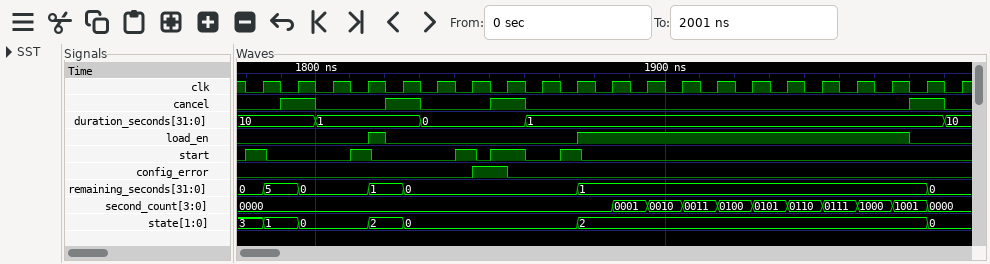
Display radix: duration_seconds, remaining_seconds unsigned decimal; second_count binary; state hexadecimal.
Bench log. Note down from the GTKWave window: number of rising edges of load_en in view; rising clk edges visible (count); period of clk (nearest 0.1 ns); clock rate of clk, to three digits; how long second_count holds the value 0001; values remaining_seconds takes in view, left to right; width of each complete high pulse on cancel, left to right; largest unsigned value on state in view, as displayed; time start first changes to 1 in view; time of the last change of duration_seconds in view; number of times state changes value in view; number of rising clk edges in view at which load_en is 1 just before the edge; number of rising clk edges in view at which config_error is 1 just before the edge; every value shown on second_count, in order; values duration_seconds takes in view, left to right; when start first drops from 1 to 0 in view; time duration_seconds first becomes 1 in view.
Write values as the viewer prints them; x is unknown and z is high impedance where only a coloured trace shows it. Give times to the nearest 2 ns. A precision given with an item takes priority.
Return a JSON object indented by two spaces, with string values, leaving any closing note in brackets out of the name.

{
  "number of rising edges of load_en in view": "2",
  "rising clk edges visible": "21",
  "period of clk": "10 ns",
  "clock rate of clk, to three digits": "100 MHz",
  "how long second_count holds the value 0001": "10 ns",
  "values remaining_seconds takes in view, left to right": "0, 5, 0, 1, 0, 1, 0",
  "width of each complete high pulse on cancel, left to right": "10 ns, 10 ns, 10 ns, 10 ns",
  "largest unsigned value on state in view, as displayed": "3",
  "time start first changes to 1 in view": "1780 ns",
  "time of the last change of duration_seconds in view": "1980 ns",
  "number of times state changes value in view": "6",
  "number of rising clk edges in view at which load_en is 1 just before the edge": "9",
  "number of rising clk edges in view at which config_error is 1 just before the edge": "1",
  "every value shown on second_count, in order": "0000, 0001, 0010, 0011, 0100, 0101, 0110, 0111, 1000, 1001, 0000",
  "values duration_seconds takes in view, left to right": "10, 1, 0, 1, 10",
  "when start first drops from 1 to 0 in view": "1786 ns",
  "time duration_seconds first becomes 1 in view": "1800 ns"
}
